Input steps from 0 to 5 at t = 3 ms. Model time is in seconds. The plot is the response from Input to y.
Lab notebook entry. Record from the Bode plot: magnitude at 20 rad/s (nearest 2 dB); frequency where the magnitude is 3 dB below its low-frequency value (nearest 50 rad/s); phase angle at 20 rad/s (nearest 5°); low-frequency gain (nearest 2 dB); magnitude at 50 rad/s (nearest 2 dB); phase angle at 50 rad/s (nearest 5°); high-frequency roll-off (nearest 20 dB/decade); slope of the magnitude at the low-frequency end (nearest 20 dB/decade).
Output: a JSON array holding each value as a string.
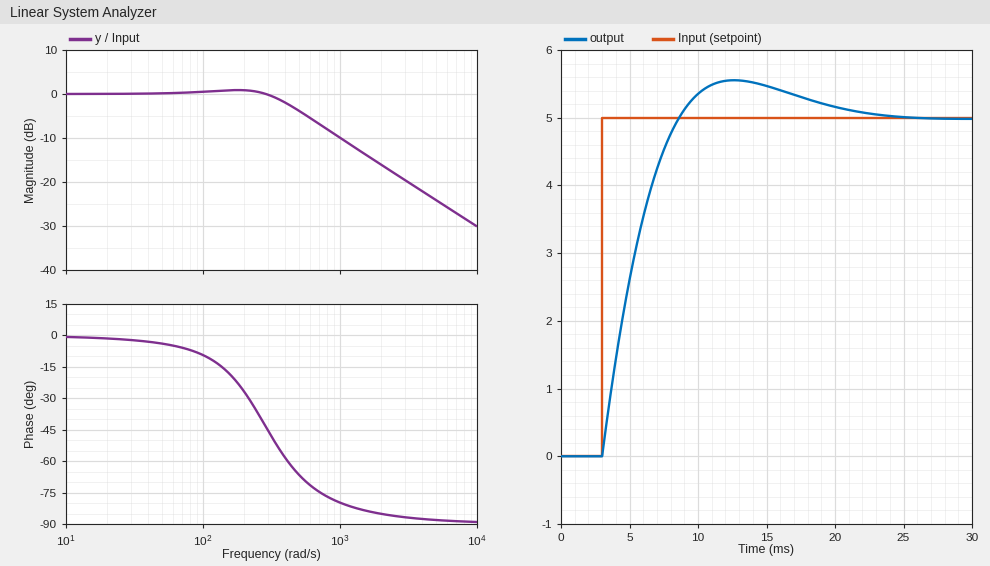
["0 dB", "450 rad/s", "0°", "0 dB", "0 dB", "-5°", "-20 dB/decade", "0 dB/decade"]
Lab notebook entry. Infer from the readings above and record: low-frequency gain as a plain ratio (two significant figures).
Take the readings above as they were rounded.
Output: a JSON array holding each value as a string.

["1.0"]
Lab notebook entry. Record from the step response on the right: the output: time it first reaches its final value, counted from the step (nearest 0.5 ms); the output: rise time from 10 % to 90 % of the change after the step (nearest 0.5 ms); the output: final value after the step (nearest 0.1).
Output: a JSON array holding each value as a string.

["5.5 ms", "4.0 ms", "5.0"]
